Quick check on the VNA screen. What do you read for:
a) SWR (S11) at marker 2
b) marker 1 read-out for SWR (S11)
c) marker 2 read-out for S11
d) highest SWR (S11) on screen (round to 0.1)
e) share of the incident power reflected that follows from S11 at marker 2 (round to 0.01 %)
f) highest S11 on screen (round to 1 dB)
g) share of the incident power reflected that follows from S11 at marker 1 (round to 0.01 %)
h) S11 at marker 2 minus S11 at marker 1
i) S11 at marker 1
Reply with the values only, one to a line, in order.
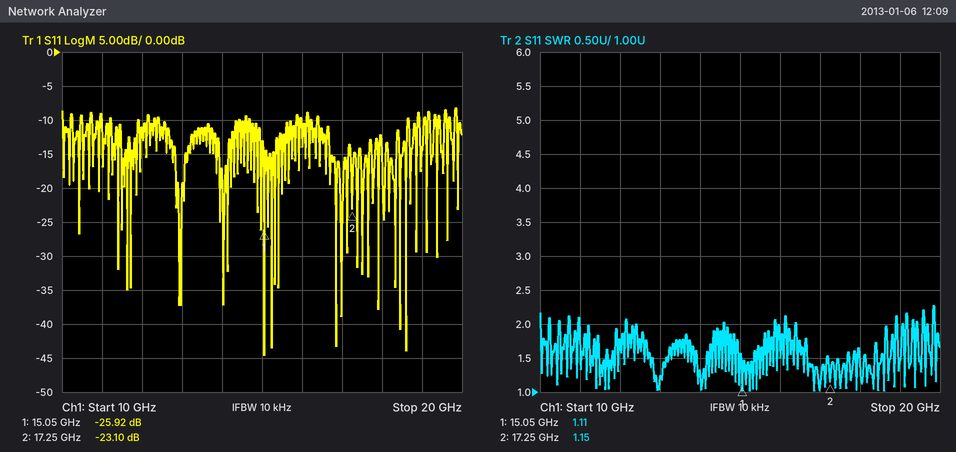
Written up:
1.15
1.11
-23.10 dB
2.3
0.49 %
-8 dB
0.26 %
2.82 dB
-25.92 dB
